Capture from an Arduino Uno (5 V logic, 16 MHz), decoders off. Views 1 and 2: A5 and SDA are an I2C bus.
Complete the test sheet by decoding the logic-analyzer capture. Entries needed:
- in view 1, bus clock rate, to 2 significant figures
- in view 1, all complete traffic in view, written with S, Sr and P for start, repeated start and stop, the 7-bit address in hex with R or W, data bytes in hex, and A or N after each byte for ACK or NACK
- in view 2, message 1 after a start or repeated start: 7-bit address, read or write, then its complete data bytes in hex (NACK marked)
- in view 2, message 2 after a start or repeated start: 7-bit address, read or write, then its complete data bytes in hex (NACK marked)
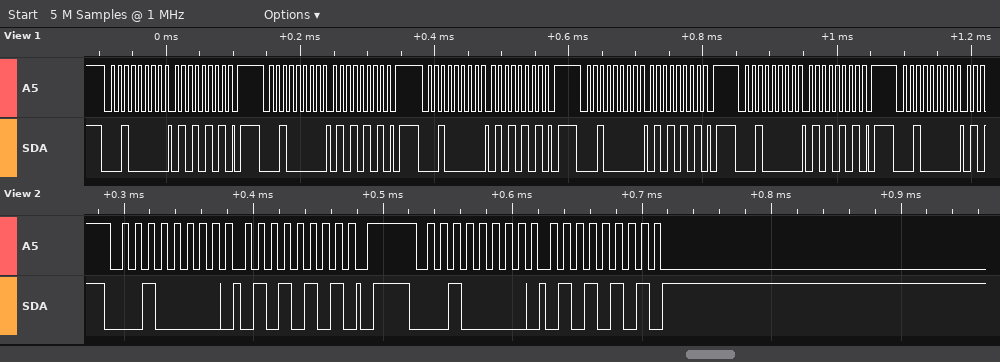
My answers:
100 kHz
S 10W A 55 A P S 10W A 55 A P S 10W A 55 A P S 10W A 55 A P S 10W A 55 A P S 10W A
0x10 write: 55
0x10 write: 55
